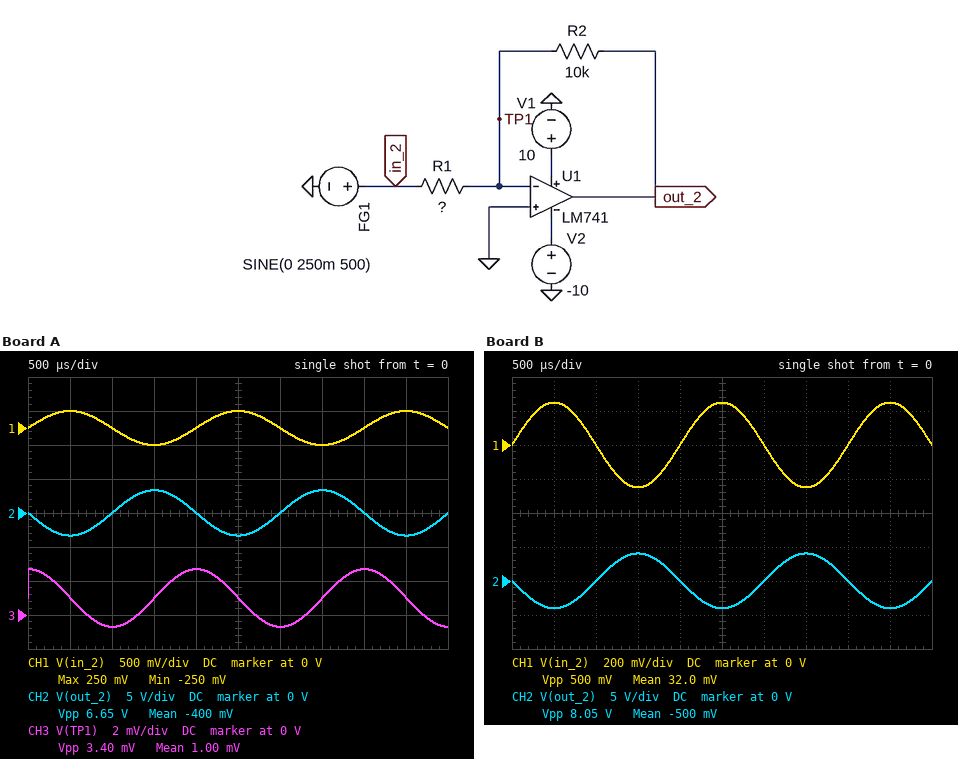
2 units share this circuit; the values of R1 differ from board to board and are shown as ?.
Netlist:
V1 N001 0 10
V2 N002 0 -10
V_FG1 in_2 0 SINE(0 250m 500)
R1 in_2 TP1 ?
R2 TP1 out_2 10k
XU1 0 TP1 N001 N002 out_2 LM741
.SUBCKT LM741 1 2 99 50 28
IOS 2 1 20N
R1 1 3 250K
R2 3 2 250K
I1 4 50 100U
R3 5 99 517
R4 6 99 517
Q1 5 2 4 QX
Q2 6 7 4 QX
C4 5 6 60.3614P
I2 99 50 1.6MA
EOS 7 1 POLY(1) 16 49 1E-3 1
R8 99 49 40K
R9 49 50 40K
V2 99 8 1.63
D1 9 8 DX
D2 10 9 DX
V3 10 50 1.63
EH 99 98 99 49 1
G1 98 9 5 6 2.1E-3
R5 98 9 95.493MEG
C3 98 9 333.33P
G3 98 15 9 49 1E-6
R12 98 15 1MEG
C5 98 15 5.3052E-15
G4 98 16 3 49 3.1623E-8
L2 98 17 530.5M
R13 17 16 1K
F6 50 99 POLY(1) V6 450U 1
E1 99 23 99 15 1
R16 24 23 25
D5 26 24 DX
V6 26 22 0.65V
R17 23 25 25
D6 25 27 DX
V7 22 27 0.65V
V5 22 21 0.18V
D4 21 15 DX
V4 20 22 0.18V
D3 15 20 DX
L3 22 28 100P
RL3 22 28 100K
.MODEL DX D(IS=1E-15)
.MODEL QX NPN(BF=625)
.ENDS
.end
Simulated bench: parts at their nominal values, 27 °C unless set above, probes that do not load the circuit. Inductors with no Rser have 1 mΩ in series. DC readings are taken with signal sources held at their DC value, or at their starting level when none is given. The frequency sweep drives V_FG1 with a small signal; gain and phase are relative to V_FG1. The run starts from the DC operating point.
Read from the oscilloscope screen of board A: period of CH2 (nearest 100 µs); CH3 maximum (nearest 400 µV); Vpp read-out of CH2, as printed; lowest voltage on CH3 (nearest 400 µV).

2.0 ms
2.8 mV
6.65 V
-800 µV
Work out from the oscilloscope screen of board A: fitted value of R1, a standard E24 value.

750 Ω
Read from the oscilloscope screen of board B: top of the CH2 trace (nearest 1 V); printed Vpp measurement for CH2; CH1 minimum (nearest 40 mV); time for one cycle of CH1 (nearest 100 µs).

4 V
8.05 V
-240 mV
2.0 ms
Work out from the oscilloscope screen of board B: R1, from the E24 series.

620 Ω
